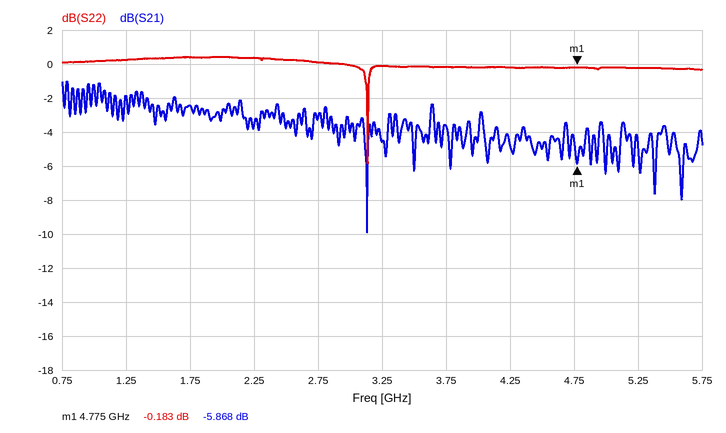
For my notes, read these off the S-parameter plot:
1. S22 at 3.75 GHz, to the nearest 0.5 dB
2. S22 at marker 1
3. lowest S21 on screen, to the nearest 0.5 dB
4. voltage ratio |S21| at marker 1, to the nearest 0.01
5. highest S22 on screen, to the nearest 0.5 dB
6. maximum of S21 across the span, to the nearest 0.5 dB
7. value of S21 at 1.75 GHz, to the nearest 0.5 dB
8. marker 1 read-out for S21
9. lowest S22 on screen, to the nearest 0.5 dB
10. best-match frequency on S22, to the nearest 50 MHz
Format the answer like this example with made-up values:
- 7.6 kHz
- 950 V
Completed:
- 0.0 dB
- -0.183 dB
- -10.0 dB
- 0.51
- 0.5 dB
- -1.0 dB
- -2.5 dB
- -5.868 dB
- -6.0 dB
- 3.15 GHz
